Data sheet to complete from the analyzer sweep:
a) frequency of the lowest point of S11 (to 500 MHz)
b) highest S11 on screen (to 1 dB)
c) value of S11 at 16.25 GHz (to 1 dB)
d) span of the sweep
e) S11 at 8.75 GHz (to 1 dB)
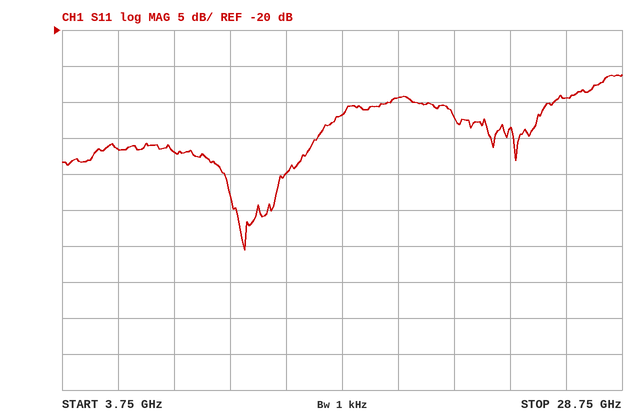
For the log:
12.0 GHz
-26 dB
-32 dB
25 GHz
-37 dB
